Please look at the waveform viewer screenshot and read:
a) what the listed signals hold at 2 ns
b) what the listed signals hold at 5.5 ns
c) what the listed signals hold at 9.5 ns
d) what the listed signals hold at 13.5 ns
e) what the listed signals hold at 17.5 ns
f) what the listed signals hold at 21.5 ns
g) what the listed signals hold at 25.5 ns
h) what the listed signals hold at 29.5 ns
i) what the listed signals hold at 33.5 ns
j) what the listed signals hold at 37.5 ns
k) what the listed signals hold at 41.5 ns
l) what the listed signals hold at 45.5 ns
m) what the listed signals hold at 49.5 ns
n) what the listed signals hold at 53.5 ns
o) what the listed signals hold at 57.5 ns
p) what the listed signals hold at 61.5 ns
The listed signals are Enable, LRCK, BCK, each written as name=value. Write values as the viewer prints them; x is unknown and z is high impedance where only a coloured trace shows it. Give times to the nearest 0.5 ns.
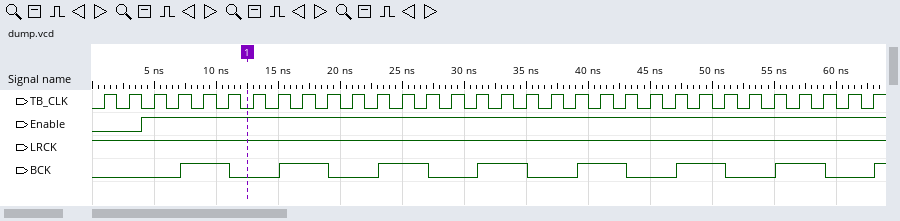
Enable=0, LRCK=1, BCK=0
Enable=1, LRCK=1, BCK=0
Enable=1, LRCK=1, BCK=1
Enable=1, LRCK=1, BCK=0
Enable=1, LRCK=1, BCK=1
Enable=1, LRCK=1, BCK=0
Enable=1, LRCK=1, BCK=1
Enable=1, LRCK=1, BCK=0
Enable=1, LRCK=1, BCK=1
Enable=1, LRCK=1, BCK=0
Enable=1, LRCK=1, BCK=1
Enable=1, LRCK=1, BCK=0
Enable=1, LRCK=1, BCK=1
Enable=1, LRCK=1, BCK=0
Enable=1, LRCK=1, BCK=1
Enable=1, LRCK=1, BCK=0
